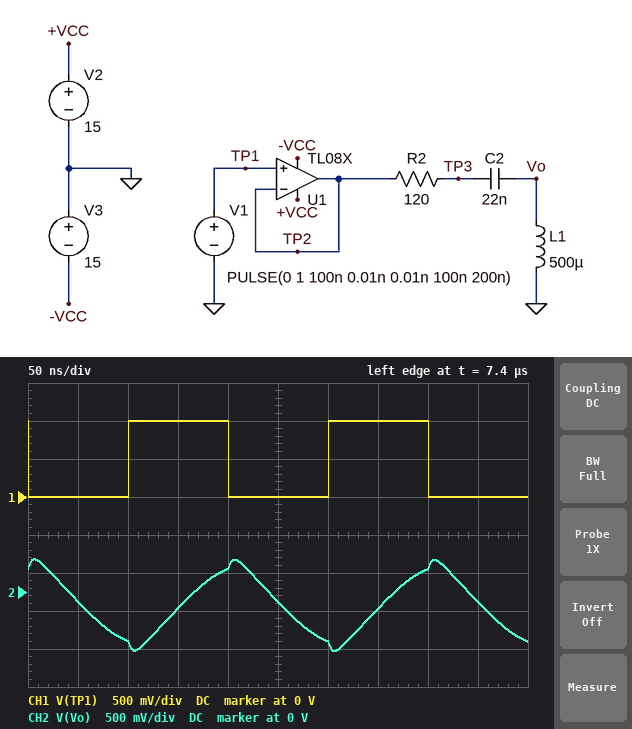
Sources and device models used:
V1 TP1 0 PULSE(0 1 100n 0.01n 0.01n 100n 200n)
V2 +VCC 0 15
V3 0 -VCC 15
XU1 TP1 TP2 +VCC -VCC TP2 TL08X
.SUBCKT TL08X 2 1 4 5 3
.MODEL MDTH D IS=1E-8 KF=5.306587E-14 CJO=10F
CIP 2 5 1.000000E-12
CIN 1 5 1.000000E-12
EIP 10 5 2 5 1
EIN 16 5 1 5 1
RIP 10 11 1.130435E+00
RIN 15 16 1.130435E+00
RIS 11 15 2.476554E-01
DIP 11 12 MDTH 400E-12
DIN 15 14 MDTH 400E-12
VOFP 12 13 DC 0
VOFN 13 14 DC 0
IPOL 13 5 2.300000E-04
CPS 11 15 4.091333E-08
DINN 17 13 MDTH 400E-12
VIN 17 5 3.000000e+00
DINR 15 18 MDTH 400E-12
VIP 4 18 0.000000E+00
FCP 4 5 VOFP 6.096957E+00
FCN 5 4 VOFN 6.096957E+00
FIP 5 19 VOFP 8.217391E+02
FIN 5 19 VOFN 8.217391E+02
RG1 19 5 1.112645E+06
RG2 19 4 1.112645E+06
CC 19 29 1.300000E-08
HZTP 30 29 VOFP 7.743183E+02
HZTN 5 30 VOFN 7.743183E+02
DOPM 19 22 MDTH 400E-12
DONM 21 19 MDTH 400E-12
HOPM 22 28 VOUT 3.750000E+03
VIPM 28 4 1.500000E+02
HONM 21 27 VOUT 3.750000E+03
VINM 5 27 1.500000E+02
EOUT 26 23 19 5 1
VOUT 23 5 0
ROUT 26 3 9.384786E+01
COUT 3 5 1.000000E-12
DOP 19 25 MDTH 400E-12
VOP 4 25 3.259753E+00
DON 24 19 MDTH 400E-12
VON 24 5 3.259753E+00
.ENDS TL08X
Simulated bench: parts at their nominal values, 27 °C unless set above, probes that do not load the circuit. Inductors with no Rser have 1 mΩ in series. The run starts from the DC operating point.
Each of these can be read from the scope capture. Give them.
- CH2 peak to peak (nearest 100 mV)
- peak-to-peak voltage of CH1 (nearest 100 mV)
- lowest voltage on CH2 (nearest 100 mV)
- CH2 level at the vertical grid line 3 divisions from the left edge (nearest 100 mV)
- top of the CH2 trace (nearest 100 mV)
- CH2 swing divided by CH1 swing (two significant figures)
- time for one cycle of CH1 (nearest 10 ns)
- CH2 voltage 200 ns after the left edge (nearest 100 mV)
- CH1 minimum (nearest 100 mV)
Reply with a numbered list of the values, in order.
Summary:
1. 1.2 V
2. 1.0 V
3. -800 mV
4. -200 mV
5. 400 mV
6. 1.2
7. 200 ns
8. 300 mV
9. 0 V
